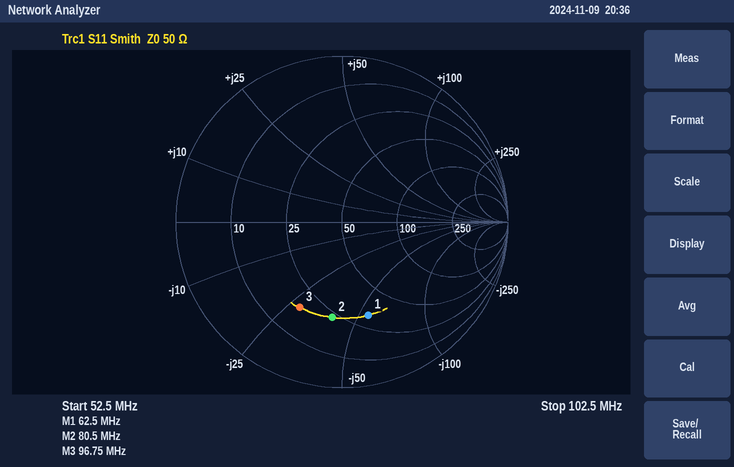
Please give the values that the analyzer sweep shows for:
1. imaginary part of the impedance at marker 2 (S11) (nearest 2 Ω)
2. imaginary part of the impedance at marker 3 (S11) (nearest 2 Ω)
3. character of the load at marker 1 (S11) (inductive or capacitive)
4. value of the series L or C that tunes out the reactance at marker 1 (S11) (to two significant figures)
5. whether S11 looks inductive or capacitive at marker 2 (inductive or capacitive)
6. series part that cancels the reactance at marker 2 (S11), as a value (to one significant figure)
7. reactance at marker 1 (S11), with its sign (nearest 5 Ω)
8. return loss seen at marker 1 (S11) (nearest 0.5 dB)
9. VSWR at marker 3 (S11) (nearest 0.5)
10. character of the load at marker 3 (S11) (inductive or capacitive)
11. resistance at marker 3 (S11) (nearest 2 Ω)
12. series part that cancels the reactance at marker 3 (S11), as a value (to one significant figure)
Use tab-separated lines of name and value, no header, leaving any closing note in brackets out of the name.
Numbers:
imaginary part of the impedance at marker 2 (S11)	-40 Ω
imaginary part of the impedance at marker 3 (S11)	-28 Ω
character of the load at marker 1 (S11)	capacitive
value of the series L or C that tunes out the reactance at marker 1 (S11)	140 nH
whether S11 looks inductive or capacitive at marker 2	capacitive
series part that cancels the reactance at marker 2 (S11), as a value	80 nH
reactance at marker 1 (S11), with its sign	-55 Ω
return loss seen at marker 1 (S11)	4.5 dB
VSWR at marker 3 (S11)	3.5
character of the load at marker 3 (S11)	capacitive
resistance at marker 3 (S11)	18 Ω
series part that cancels the reactance at marker 3 (S11), as a value	50 nH
